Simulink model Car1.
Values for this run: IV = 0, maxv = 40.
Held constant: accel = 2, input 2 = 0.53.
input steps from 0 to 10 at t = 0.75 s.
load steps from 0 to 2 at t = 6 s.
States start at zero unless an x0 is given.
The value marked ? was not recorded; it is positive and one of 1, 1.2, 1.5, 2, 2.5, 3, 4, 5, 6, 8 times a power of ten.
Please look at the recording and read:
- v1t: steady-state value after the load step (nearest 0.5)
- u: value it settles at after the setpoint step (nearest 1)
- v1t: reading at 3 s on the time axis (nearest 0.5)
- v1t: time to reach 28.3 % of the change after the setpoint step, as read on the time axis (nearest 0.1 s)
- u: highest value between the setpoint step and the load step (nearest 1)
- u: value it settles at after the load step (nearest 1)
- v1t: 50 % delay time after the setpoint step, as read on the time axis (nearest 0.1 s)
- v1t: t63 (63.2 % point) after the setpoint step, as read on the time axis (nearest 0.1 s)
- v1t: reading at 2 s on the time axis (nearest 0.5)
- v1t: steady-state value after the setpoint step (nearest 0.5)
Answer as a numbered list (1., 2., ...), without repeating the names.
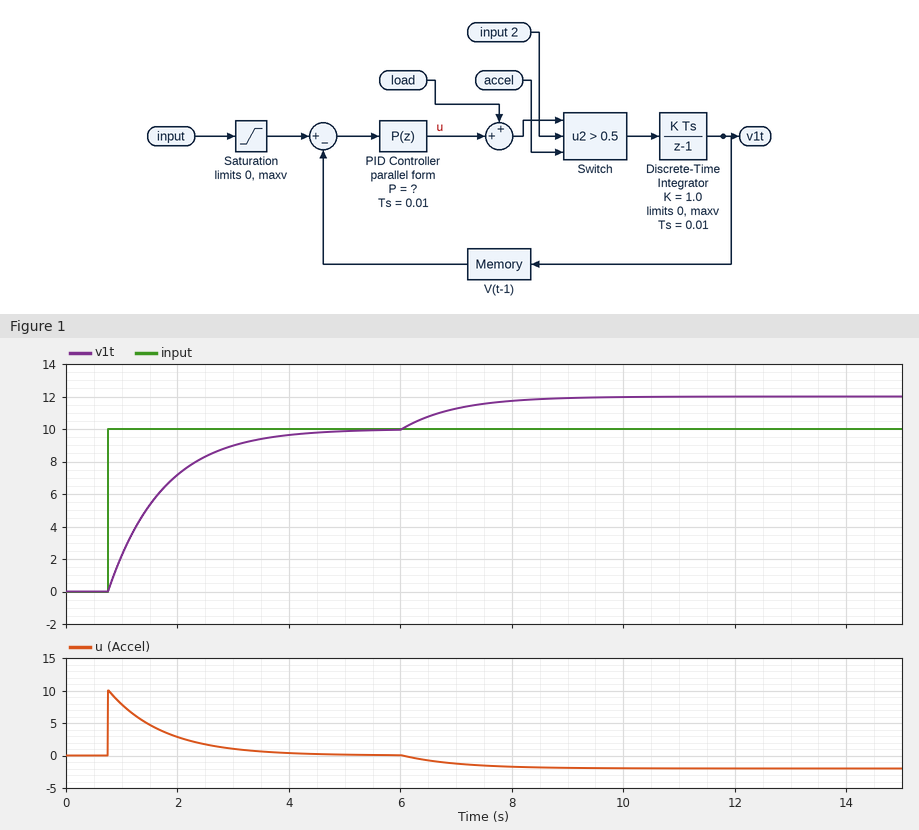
1. 12.0
2. 0
3. 9.0
4. 1.1 s
5. 10
6. -2
7. 1.4 s
8. 1.7 s
9. 7.0
10. 10.0
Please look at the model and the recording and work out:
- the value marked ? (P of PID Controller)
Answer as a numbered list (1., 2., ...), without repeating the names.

1. 1
